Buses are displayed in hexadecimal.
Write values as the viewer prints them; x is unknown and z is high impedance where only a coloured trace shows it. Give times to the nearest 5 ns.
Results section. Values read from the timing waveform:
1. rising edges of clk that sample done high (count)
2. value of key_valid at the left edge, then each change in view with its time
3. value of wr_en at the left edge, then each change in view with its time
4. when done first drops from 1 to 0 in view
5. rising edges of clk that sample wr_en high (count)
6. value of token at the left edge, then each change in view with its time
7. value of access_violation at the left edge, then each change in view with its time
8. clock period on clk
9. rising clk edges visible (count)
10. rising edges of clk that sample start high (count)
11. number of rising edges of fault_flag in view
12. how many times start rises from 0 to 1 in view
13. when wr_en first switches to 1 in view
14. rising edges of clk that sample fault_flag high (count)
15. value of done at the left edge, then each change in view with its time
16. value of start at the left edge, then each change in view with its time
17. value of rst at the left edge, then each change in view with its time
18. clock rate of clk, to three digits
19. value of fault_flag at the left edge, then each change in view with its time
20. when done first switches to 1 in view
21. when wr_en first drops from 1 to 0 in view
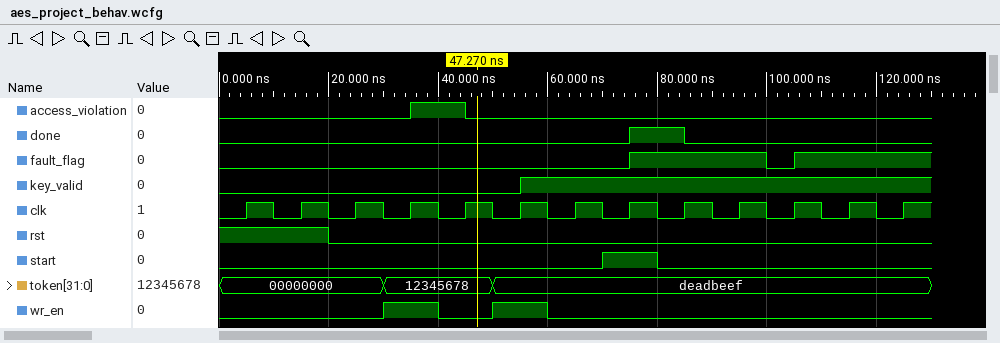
1
0, 1 at 55 ns
0, 1 at 30 ns, 0 at 40 ns, 1 at 50 ns, 0 at 60 ns
85 ns
2
00000000, 12345678 at 30 ns, deadbeef at 50 ns
0, 1 at 35 ns, 0 at 45 ns
10 ns
13
1
2
1
30 ns
4
0, 1 at 75 ns, 0 at 85 ns
0, 1 at 70 ns, 0 at 80 ns
1, 0 at 20 ns
100 MHz
0, 1 at 75 ns, 0 at 100 ns, 1 at 105 ns
75 ns
40 ns
